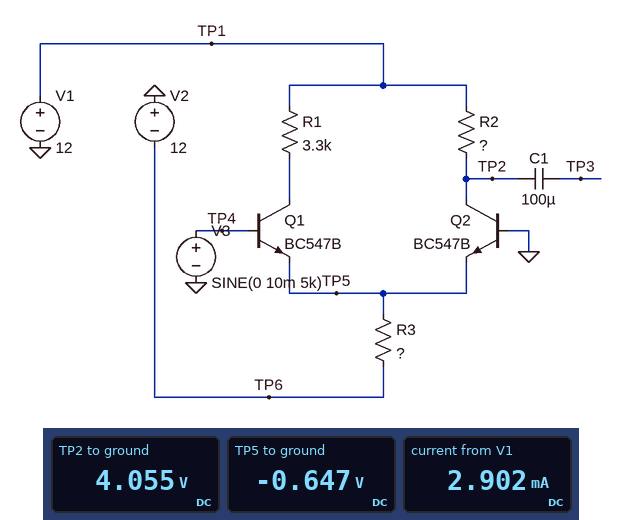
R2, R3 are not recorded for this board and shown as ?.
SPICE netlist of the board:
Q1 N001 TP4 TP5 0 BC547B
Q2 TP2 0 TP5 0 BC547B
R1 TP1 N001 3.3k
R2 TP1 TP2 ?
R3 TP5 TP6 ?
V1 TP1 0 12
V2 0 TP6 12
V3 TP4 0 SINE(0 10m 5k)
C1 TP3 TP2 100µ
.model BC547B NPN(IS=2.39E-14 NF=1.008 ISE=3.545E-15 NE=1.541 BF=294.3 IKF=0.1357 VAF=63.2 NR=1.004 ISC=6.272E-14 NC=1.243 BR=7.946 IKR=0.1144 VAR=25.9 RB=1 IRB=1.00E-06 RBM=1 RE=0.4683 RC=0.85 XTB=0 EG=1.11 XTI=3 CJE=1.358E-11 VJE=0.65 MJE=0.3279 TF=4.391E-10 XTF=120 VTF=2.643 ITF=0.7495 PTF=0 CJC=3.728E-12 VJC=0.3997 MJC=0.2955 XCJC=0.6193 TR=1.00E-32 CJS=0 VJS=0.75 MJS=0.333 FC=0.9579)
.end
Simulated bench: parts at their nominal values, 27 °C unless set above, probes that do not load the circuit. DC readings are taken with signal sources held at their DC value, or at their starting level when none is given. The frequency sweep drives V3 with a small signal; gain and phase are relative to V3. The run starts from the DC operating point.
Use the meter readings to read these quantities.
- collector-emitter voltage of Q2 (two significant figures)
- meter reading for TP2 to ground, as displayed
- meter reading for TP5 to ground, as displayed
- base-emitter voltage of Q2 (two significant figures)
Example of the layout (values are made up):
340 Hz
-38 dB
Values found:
4.7 V
4.055 V
-0.647 V
650 mV
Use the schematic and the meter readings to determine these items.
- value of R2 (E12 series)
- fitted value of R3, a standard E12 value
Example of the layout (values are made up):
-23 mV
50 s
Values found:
5.6 kΩ
3.9 kΩ
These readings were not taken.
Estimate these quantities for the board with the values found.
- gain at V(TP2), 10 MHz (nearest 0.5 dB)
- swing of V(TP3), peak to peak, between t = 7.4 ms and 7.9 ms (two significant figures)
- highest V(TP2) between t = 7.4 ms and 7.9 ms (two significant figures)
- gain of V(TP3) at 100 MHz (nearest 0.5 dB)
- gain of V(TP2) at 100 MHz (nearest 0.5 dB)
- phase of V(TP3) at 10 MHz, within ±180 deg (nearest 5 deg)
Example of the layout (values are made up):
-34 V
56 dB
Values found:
41.5 dB
2.7 V
5.4 V
27.0 dB
27.0 dB
-30 deg
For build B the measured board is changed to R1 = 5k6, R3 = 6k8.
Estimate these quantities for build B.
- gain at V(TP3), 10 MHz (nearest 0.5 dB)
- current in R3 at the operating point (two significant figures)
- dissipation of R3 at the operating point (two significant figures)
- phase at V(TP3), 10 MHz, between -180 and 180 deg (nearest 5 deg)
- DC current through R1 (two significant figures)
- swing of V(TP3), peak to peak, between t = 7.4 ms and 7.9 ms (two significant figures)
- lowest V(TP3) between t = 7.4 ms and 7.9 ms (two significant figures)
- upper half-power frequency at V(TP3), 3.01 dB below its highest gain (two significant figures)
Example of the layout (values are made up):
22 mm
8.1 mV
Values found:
37.0 dB
1.7 mA
19 mW
-30 deg
830 µA
1.6 V
-810 mV
19 MHz
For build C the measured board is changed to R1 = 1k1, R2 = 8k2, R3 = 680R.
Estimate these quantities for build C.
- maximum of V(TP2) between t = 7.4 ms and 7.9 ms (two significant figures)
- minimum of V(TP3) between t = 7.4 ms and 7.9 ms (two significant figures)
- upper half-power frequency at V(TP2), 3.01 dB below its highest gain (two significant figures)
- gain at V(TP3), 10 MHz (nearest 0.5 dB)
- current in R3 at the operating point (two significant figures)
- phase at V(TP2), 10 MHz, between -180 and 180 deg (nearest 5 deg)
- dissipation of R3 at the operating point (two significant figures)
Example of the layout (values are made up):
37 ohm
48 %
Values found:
-710 mV
-4.3 mV
400 MHz
-6.5 dB
17 mA
0 deg
190 mW
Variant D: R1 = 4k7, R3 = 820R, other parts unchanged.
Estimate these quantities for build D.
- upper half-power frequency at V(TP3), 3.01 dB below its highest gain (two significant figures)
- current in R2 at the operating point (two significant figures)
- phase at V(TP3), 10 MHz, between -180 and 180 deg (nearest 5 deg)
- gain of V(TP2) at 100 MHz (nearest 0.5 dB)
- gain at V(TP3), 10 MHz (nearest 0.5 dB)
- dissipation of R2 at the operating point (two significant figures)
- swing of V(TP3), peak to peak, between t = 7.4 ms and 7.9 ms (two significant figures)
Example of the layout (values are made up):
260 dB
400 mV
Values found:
450 MHz
2.3 mA
0 deg
-7.5 dB
-6.5 dB
29 mW
9.5 mV
